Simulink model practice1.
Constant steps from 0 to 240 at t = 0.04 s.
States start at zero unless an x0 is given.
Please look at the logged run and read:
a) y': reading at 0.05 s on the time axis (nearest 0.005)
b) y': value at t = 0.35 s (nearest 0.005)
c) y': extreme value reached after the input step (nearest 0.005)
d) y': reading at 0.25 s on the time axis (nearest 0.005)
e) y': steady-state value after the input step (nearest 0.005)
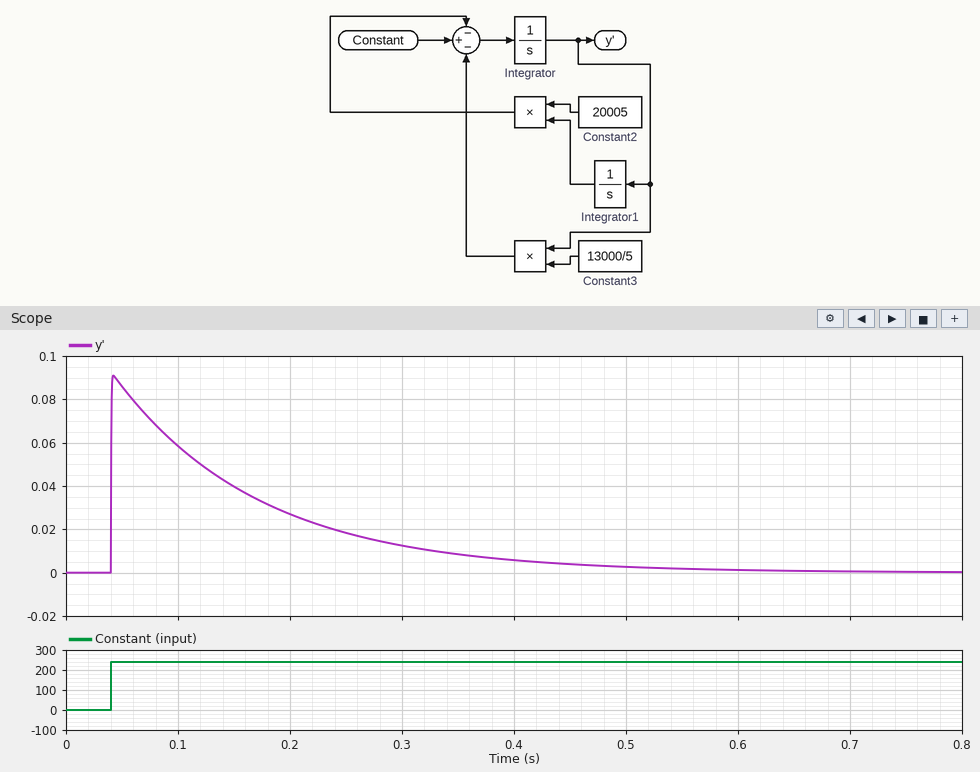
0.085
0.010
0.090
0.020
0.000
